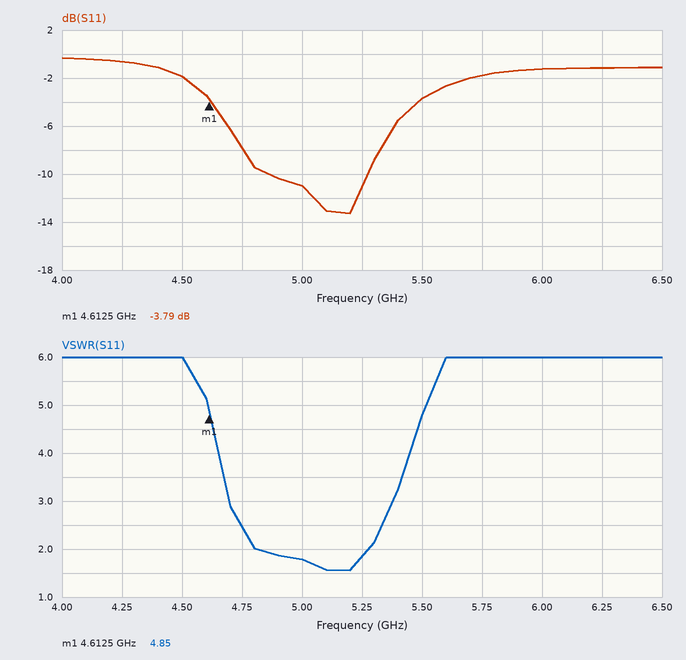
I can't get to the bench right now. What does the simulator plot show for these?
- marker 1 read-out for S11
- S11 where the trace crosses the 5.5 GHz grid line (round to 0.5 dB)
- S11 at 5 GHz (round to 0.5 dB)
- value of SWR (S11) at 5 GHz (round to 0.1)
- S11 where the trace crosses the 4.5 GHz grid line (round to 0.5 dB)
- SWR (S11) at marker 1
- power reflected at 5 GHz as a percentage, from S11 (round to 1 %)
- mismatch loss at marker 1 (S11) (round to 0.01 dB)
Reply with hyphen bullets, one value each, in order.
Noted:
- -3.79 dB
- -3.5 dB
- -11.0 dB
- 1.8
- -2.0 dB
- 4.85
- 8 %
- 2.35 dB
